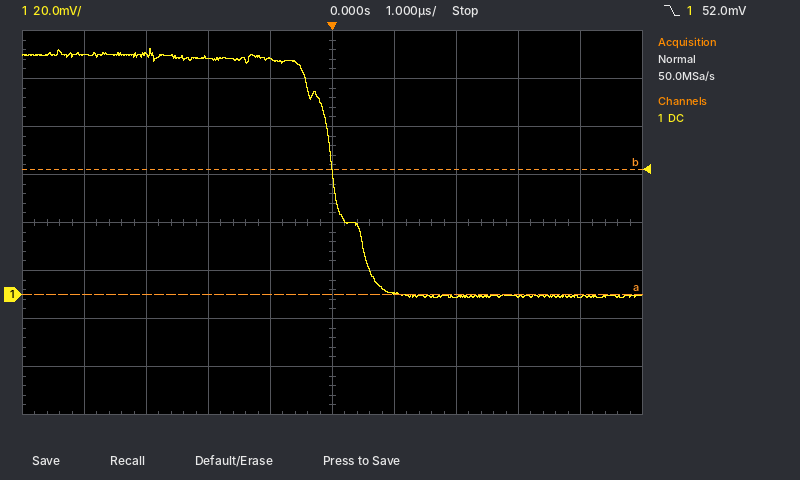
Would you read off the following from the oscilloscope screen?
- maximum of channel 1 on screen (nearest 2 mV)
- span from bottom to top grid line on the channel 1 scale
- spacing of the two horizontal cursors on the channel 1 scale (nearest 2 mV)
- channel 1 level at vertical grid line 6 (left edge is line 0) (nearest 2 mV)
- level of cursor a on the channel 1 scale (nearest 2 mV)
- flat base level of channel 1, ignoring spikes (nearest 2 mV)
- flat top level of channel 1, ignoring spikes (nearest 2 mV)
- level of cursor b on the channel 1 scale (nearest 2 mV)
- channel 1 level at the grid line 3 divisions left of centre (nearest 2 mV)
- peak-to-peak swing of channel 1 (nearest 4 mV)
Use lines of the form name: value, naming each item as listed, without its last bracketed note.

maximum of channel 1 on screen: 102 mV
span from bottom to top grid line on the channel 1 scale: 160 mV
spacing of the two horizontal cursors on the channel 1 scale: 52 mV
channel 1 level at vertical grid line 6 (left edge is line 0): 0 mV
level of cursor a on the channel 1 scale: 0 mV
flat base level of channel 1, ignoring spikes: 0 mV
flat top level of channel 1, ignoring spikes: 100 mV
level of cursor b on the channel 1 scale: 52 mV
channel 1 level at the grid line 3 divisions left of centre: 100 mV
peak-to-peak swing of channel 1: 104 mV
